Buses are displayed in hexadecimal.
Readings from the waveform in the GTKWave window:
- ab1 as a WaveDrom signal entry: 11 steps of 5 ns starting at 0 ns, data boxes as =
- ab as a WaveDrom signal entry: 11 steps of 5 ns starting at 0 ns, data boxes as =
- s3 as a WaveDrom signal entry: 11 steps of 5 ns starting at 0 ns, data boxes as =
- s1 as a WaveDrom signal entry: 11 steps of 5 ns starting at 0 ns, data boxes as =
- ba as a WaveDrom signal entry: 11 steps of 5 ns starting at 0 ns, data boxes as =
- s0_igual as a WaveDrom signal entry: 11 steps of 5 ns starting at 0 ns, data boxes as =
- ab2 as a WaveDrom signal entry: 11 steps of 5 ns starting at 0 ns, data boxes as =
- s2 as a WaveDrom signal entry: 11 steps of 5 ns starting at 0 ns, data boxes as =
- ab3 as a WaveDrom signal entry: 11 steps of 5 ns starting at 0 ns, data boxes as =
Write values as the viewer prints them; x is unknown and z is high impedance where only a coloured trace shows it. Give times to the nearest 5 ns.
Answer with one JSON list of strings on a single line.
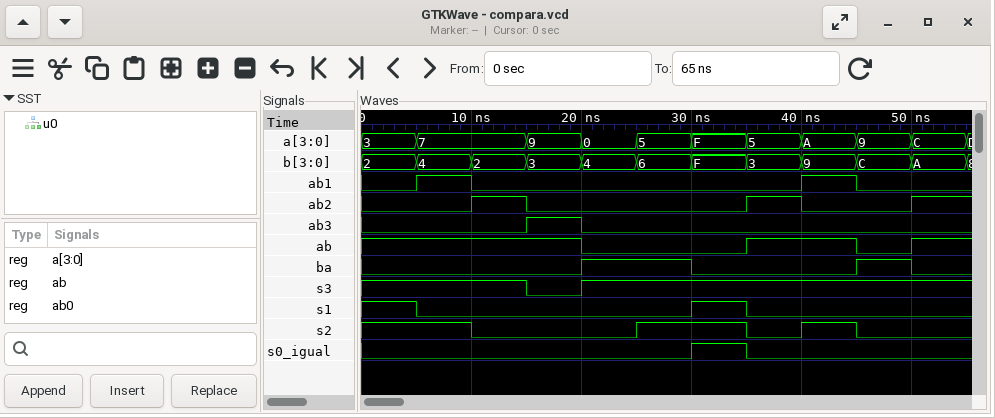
["{name: 'ab1', wave: '010.....10.'}", "{name: 'ab', wave: '1...0..1.01'}", "{name: 's3', wave: '1..01......'}", "{name: 's1', wave: '10....10...'}", "{name: 'ba', wave: '0...1.0..10'}", "{name: 's0_igual', wave: '0.....10...'}", "{name: 'ab2', wave: '0.10...10.1'}", "{name: 's2', wave: '1.0..1.010.'}", "{name: 'ab3', wave: '0..10......'}"]
